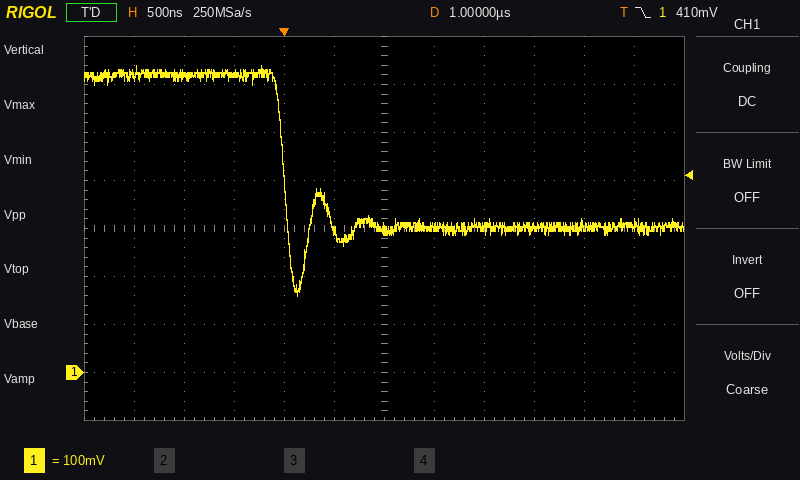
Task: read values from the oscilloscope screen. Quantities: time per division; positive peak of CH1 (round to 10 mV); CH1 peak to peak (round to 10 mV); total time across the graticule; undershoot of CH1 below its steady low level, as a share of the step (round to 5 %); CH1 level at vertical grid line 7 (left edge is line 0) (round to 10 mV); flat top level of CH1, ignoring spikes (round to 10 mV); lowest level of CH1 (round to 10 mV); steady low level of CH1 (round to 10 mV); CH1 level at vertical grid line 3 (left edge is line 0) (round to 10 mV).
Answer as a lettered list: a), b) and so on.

a) 500 ns
b) 640 mV
c) 480 mV
d) 6 µs
e) 45 %
f) 300 mV
g) 620 mV
h) 160 mV
i) 300 mV
j) 620 mV
